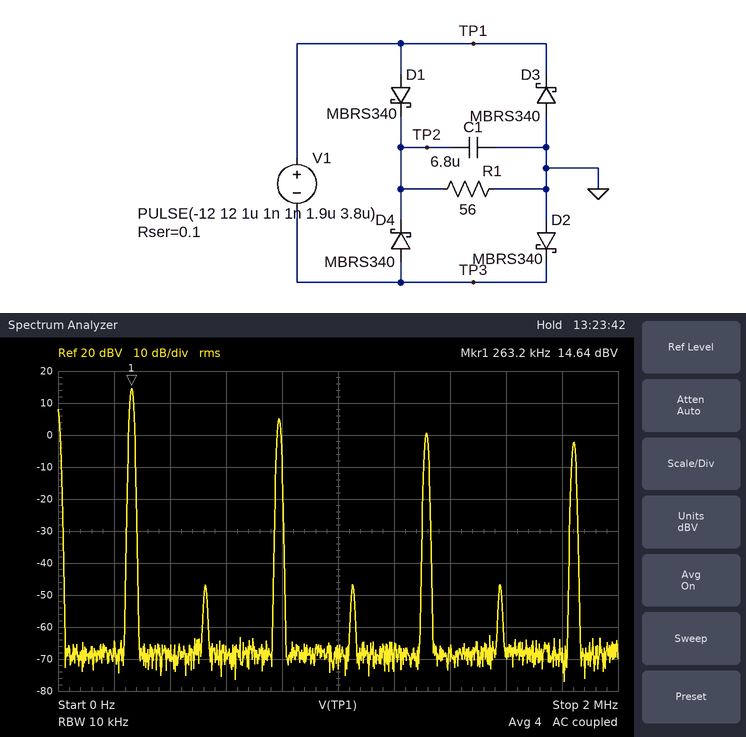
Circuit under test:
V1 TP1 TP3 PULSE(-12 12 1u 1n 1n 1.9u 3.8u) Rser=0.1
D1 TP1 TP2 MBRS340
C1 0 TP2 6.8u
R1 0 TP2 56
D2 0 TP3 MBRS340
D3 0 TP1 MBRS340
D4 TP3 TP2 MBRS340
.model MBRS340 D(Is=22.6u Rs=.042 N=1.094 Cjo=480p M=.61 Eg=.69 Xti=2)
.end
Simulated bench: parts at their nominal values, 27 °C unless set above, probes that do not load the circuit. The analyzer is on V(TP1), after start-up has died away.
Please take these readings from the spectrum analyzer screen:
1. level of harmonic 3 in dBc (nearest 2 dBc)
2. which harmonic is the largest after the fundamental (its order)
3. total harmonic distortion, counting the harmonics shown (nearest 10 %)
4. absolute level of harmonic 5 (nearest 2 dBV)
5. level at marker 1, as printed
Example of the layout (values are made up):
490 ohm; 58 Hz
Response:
-10 dBc; 3; 40 %; 0 dBV; 14.64 dBV
